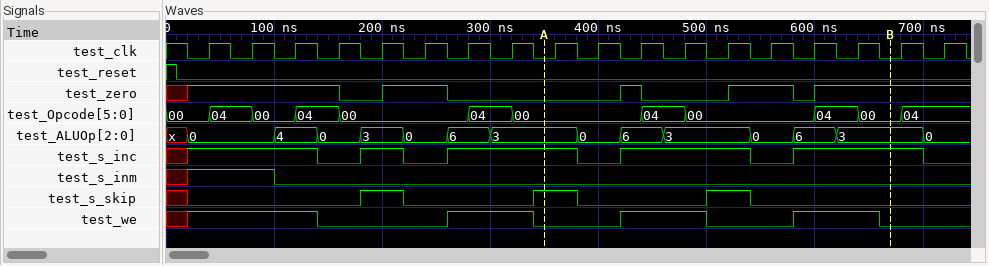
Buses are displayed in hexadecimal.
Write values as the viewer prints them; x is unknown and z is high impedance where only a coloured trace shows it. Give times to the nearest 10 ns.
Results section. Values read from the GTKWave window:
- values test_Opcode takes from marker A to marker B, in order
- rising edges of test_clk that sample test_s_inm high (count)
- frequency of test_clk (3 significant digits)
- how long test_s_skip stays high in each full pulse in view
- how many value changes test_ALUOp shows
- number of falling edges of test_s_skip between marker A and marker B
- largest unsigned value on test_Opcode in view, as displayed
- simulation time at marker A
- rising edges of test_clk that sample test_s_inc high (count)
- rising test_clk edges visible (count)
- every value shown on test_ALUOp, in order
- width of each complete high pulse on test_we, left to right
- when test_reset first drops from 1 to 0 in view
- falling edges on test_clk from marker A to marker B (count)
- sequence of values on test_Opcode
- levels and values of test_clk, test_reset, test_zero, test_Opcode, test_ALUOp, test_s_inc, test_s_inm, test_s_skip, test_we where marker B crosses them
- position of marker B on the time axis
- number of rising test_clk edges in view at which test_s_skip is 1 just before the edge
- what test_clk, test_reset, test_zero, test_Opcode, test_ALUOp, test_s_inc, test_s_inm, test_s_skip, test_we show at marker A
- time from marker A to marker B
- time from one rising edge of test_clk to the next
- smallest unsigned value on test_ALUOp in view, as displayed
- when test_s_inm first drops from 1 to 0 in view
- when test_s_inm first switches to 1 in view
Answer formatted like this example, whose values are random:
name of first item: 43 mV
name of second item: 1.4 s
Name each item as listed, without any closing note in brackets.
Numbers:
values test_Opcode takes from marker A to marker B, in order: 00, 04, 00, 04, 00
rising edges of test_clk that sample test_s_inm high: 2
frequency of test_clk: 25.0 MHz
how long test_s_skip stays high in each full pulse in view: 40 ns, 40 ns, 40 ns
how many value changes test_ALUOp shows: 14
number of falling edges of test_s_skip between marker A and marker B: 2
largest unsigned value on test_Opcode in view, as displayed: 04
simulation time at marker A: 350 ns
rising edges of test_clk that sample test_s_inc high: 13
rising test_clk edges visible: 18
every value shown on test_ALUOp, in order: x, 0, 4, 0, 3, 0, 6, 3, 0, 6, 3, 0, 6, 3, 0
width of each complete high pulse on test_we, left to right: 80 ns, 80 ns, 80 ns
when test_reset first drops from 1 to 0 in view: 10 ns
falling edges on test_clk from marker A to marker B: 8
sequence of values on test_Opcode: 00, 04, 00, 04, 00, 04, 00, 04, 00, 04, 00, 04
levels and values of test_clk, test_reset, test_zero, test_Opcode, test_ALUOp, test_s_inc, test_s_inm, test_s_skip, test_we where marker B crosses them: test_clk=0, test_reset=0, test_zero=1, test_Opcode=00, test_ALUOp=3, test_s_inc=1, test_s_inm=0, test_s_skip=0, test_we=0
position of marker B on the time axis: 670 ns
number of rising test_clk edges in view at which test_s_skip is 1 just before the edge: 3
what test_clk, test_reset, test_zero, test_Opcode, test_ALUOp, test_s_inc, test_s_inm, test_s_skip, test_we show at marker A: test_clk=0, test_reset=0, test_zero=0, test_Opcode=00, test_ALUOp=3, test_s_inc=1, test_s_inm=0, test_s_skip=1, test_we=0
time from marker A to marker B: 320 ns
time from one rising edge of test_clk to the next: 40 ns
smallest unsigned value on test_ALUOp in view, as displayed: 0
when test_s_inm first drops from 1 to 0 in view: 100 ns
when test_s_inm first switches to 1 in view: 20 ns
